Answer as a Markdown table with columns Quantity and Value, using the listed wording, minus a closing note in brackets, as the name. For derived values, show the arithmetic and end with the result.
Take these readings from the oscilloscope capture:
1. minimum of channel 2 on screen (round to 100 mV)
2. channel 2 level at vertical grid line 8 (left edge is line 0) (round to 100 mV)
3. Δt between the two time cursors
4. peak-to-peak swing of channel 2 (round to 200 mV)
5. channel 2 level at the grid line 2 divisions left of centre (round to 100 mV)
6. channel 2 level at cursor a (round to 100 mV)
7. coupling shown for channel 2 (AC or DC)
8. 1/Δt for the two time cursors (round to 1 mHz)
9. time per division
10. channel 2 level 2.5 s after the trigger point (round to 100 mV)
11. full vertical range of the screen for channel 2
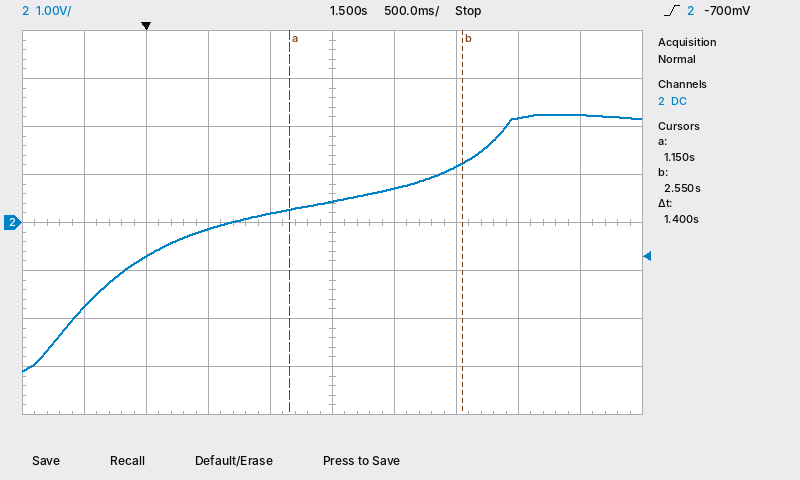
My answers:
| Quantity | Value |
|---|---|
| minimum of channel 2 on screen | -3.1 V |
| channel 2 level at vertical grid line 8 (left edge is line 0) | 2.2 V |
| Δt between the two time cursors | 1.4 s |
| peak-to-peak swing of channel 2 | 5.4 V |
| channel 2 level at the grid line 2 divisions left of centre | -100 mV |
| channel 2 level at cursor a | 300 mV |
| coupling shown for channel 2 | DC |
| 1/Δt for the two time cursors | 1 / 1.4 s ≈ 714 mHz |
| time per division | 500 ms |
| channel 2 level 2.5 s after the trigger point | 1.2 V |
| full vertical range of the screen for channel 2 | 8 V |
